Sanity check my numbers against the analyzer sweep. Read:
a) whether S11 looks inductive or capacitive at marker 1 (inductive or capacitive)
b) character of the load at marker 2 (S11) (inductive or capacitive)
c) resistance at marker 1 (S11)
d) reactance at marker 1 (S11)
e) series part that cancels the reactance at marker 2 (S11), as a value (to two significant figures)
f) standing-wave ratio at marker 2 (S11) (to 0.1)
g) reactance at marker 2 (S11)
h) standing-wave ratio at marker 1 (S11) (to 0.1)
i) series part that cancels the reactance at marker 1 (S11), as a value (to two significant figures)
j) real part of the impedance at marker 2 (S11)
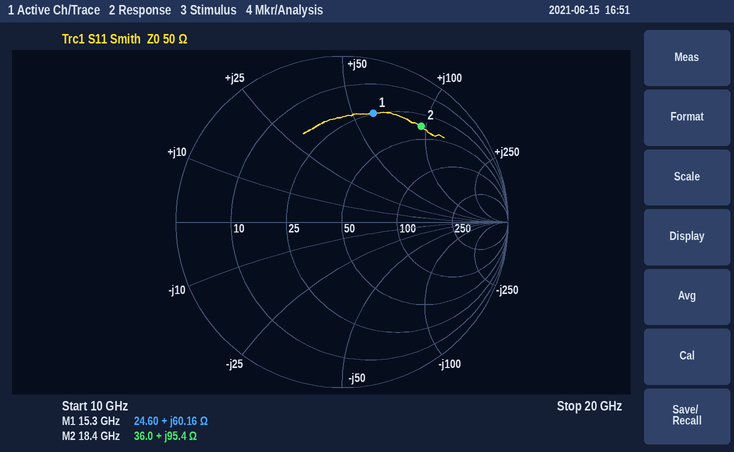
inductive
inductive
24.60 Ω
+60.16 Ω
91 fF
7.0
+95.4 Ω
5.3
170 fF
36.0 Ω
